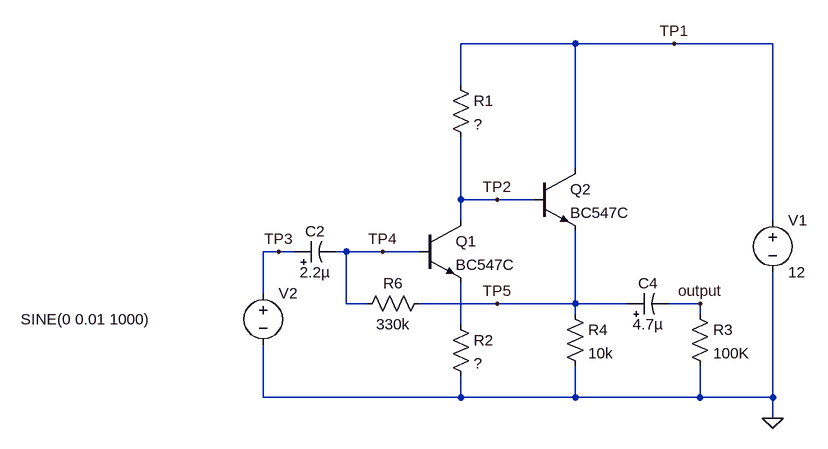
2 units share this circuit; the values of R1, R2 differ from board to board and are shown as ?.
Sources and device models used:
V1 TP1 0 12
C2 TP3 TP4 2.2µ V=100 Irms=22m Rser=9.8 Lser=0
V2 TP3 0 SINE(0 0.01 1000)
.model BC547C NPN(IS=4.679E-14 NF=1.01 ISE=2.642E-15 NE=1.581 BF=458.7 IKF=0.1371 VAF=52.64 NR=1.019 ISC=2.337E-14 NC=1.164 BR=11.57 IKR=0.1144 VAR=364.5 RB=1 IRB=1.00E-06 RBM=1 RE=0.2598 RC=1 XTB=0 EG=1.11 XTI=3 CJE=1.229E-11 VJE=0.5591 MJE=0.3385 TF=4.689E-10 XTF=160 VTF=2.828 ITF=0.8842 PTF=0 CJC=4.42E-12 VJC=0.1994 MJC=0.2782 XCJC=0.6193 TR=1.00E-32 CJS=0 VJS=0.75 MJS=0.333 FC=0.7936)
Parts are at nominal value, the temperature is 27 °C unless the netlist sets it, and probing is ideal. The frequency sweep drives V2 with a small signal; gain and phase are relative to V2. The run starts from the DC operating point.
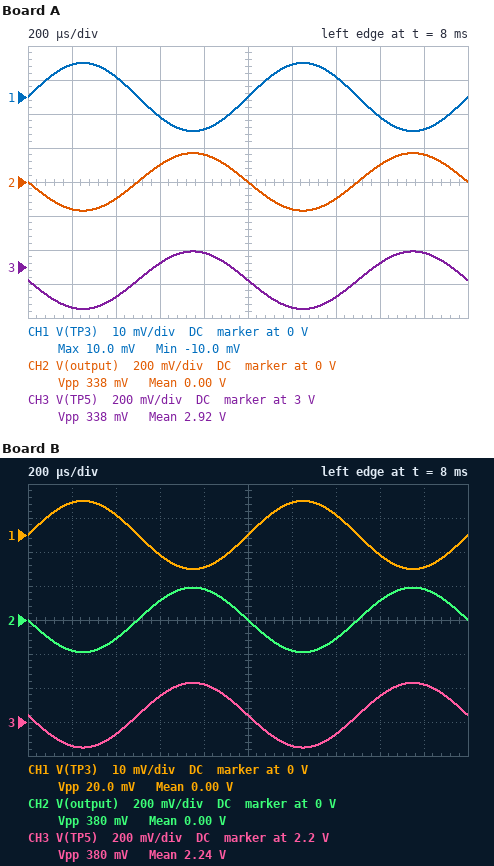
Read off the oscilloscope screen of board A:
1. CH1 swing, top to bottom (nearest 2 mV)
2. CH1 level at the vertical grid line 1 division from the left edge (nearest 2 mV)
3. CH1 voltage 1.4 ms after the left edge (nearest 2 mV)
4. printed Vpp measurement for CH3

20 mV
10 mV
6 mV
338 mV
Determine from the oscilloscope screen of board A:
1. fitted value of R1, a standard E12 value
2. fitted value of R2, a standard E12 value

3.3 kΩ
180 Ω
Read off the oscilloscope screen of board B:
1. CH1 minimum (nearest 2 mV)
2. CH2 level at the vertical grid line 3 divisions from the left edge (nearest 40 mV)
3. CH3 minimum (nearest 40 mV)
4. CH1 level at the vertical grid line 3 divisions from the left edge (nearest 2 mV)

-10 mV
120 mV
2.04 V
-6 mV
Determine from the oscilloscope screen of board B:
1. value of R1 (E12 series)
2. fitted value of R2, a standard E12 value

5.6 kΩ
270 Ω
